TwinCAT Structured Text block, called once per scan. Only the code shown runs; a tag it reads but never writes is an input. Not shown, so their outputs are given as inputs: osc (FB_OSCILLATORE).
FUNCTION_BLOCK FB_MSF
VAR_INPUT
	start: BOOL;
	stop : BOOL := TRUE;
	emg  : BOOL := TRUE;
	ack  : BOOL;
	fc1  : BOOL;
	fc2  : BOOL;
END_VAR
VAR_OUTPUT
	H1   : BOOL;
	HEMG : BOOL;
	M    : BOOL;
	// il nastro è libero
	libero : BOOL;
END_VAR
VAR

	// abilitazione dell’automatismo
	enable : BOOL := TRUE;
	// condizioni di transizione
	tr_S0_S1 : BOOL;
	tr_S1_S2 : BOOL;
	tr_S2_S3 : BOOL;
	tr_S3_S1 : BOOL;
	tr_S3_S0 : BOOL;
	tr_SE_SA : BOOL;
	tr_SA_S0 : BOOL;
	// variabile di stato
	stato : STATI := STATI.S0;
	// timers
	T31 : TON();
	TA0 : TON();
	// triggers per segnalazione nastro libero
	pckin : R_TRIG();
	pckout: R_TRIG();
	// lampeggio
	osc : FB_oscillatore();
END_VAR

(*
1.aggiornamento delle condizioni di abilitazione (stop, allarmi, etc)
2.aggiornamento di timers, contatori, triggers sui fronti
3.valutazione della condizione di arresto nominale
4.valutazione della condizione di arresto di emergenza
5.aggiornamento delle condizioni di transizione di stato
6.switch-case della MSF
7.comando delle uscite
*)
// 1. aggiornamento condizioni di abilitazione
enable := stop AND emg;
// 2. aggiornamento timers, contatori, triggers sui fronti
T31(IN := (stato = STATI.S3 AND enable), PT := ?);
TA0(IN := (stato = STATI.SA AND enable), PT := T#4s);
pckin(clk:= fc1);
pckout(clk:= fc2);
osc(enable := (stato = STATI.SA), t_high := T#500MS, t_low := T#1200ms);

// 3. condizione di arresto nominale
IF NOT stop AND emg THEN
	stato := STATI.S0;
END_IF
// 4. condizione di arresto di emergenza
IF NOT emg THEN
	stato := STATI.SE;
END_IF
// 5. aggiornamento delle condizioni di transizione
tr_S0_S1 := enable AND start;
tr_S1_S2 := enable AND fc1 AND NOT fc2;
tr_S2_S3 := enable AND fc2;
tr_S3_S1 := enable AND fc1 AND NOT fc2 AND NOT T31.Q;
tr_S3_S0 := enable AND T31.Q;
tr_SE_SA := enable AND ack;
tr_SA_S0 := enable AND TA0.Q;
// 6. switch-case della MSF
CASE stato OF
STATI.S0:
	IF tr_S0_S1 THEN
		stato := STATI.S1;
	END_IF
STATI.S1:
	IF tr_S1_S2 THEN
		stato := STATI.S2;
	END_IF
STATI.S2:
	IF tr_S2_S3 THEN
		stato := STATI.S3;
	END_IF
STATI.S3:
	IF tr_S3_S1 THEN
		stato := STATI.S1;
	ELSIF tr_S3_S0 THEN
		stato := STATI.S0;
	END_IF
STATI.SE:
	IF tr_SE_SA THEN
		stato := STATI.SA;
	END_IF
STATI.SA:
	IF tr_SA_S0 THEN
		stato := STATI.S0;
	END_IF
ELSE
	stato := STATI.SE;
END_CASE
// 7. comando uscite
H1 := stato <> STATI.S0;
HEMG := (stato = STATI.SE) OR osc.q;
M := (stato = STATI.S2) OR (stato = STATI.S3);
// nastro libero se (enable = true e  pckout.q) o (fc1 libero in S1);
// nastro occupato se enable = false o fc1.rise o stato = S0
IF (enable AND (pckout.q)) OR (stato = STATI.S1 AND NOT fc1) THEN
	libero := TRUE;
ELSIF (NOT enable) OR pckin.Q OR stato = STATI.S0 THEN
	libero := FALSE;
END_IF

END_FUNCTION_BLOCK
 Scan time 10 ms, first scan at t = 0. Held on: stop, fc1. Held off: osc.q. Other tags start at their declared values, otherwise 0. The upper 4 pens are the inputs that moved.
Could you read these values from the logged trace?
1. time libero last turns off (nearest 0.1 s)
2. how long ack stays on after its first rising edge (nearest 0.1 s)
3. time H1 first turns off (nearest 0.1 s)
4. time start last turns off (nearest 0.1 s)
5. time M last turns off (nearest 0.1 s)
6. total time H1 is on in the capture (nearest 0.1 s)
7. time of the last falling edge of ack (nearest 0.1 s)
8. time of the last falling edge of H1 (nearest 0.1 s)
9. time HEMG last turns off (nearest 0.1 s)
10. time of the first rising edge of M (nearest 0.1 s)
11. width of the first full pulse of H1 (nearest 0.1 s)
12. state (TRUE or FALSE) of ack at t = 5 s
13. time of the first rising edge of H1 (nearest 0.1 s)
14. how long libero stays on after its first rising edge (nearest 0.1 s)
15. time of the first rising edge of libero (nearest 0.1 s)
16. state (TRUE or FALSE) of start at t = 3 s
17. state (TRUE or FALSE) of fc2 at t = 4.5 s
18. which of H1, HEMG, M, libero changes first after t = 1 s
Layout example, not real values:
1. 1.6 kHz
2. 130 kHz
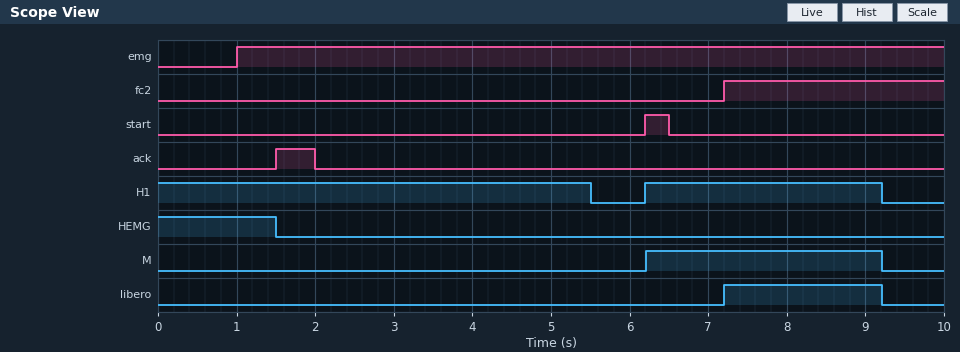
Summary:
1. 9.2 s
2. 0.5 s
3. 5.5 s
4. 6.5 s
5. 9.2 s
6. 8.5 s
7. 2.0 s
8. 9.2 s
9. 1.5 s
10. 6.2 s
11. 3.0 s
12. FALSE
13. 6.2 s
14. 2.0 s
15. 7.2 s
16. FALSE
17. FALSE
18. HEMG
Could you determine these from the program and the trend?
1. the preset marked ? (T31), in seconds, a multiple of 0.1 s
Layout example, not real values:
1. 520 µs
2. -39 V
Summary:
1. 2.0 s
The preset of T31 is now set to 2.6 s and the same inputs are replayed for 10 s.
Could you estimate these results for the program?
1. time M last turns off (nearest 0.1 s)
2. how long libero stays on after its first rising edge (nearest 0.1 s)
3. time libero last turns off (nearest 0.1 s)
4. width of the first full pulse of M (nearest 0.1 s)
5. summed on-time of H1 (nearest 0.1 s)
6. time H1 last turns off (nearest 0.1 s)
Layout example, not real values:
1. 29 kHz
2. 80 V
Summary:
1. 9.8 s
2. 2.6 s
3. 9.8 s
4. 3.6 s
5. 9.1 s
6. 9.8 s
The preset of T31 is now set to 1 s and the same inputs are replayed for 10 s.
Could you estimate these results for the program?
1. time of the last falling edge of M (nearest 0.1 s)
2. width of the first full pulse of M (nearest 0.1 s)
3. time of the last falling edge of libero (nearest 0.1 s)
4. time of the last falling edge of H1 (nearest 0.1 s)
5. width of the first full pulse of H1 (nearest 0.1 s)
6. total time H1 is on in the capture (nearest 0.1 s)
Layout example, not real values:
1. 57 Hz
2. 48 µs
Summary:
1. 8.2 s
2. 2.0 s
3. 8.2 s
4. 8.2 s
5. 2.0 s
6. 7.5 s
